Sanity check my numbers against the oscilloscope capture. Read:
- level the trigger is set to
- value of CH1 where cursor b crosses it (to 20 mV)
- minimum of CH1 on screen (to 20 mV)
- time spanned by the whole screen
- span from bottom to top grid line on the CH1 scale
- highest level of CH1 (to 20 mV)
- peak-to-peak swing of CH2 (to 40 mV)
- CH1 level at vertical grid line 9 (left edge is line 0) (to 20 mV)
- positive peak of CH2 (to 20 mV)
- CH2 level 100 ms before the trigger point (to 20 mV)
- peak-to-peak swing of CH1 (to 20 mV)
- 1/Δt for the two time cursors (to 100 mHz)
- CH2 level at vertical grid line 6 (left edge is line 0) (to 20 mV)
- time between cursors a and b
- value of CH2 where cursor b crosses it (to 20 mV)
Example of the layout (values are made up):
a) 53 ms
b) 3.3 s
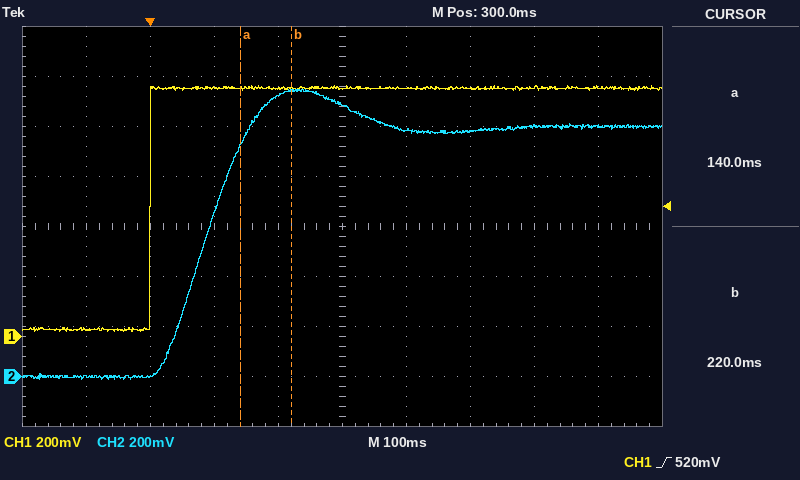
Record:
a) 520 mV
b) 1.00 V
c) 20 mV
d) 1 s
e) 1.6 V
f) 1.00 V
g) 1.16 V
h) 1.00 V
i) 1.14 V
j) 0 mV
k) 980 mV
l) 12.5 Hz
m) 980 mV
n) 80 ms
o) 1.14 V
